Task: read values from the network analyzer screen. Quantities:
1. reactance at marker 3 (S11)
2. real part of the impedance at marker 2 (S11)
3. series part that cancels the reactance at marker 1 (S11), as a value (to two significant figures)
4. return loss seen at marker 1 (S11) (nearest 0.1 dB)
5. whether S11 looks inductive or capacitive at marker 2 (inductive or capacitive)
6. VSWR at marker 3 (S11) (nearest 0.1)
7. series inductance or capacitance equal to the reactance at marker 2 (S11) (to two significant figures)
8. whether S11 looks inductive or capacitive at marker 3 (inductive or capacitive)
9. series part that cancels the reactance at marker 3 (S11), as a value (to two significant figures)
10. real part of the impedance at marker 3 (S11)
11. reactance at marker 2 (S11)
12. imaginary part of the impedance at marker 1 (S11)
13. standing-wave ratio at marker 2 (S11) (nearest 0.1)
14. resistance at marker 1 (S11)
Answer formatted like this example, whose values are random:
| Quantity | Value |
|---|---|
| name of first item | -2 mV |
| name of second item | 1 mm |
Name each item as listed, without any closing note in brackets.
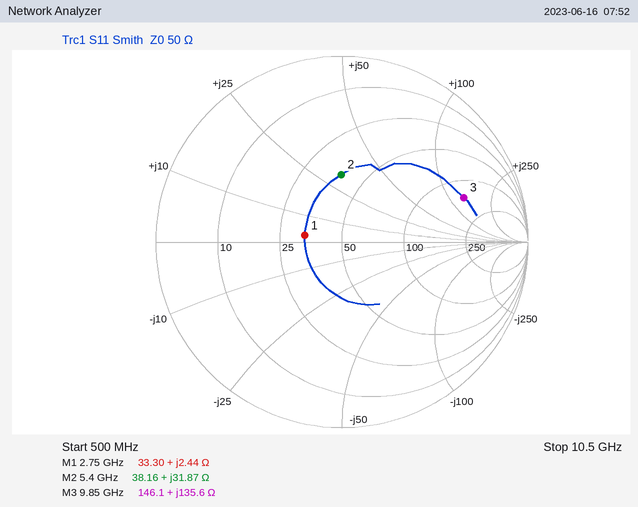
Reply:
| Quantity | Value |
|---|---|
| reactance at marker 3 | +135.6 Ω |
| real part of the impedance at marker 2 | 38.16 Ω |
| series part that cancels the reactance at marker 1 (S11), as a value | 24 pF |
| return loss seen at marker 1 (S11) | 13.9 dB |
| whether S11 looks inductive or capacitive at marker 2 | inductive |
| VSWR at marker 3 (S11) | 5.6 |
| series inductance or capacitance equal to the reactance at marker 2 (S11) | 940 pH |
| whether S11 looks inductive or capacitive at marker 3 | inductive |
| series part that cancels the reactance at marker 3 (S11), as a value | 120 fF |
| real part of the impedance at marker 3 | 146.1 Ω |
| reactance at marker 2 | +31.87 Ω |
| imaginary part of the impedance at marker 1 | +2.44 Ω |
| standing-wave ratio at marker 2 (S11) | 2.1 |
| resistance at marker 1 | 33.30 Ω |
